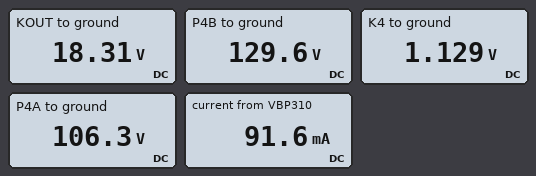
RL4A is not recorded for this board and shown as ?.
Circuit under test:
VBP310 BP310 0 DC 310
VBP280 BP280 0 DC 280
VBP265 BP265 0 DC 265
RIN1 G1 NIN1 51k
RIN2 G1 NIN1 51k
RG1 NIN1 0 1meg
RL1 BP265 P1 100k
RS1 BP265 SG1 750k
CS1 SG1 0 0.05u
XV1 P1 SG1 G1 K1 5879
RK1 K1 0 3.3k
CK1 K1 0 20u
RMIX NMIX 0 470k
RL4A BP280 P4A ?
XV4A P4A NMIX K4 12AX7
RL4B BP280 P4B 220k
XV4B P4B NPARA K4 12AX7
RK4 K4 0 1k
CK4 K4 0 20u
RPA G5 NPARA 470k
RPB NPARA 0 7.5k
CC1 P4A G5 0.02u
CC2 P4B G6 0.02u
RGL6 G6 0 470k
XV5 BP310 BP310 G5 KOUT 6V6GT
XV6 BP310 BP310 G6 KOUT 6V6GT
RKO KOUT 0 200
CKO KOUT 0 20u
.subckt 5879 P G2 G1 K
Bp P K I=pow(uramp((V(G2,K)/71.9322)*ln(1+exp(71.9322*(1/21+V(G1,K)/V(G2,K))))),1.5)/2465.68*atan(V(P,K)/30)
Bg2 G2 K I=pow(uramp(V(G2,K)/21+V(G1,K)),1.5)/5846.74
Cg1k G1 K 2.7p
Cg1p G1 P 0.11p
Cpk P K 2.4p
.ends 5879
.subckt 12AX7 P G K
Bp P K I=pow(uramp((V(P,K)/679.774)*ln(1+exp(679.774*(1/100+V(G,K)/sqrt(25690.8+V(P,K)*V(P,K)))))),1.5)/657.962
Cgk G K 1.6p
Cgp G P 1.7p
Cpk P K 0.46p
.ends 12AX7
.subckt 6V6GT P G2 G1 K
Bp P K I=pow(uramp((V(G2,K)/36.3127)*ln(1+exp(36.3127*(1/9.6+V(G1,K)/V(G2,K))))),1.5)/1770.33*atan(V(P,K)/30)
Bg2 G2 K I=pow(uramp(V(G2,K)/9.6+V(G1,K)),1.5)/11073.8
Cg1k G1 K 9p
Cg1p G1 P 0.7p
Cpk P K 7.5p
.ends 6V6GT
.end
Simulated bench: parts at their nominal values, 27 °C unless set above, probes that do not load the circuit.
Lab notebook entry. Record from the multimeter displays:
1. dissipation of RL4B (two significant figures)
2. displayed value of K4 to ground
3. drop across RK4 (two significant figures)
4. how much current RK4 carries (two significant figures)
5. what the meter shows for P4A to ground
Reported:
100 mW
1.129 V
1.1 V
1.1 mA
106.3 V
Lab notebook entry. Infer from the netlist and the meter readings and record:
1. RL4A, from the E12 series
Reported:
390 kΩ
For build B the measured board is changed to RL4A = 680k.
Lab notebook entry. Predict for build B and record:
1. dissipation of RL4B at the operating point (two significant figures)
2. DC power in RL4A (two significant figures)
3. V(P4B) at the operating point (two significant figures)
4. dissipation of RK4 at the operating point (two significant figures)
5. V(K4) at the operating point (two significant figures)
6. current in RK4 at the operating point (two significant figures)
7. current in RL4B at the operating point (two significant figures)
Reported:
110 mW
60 mW
120 V
1.0 mW
1.0 V
1.0 mA
720 µA
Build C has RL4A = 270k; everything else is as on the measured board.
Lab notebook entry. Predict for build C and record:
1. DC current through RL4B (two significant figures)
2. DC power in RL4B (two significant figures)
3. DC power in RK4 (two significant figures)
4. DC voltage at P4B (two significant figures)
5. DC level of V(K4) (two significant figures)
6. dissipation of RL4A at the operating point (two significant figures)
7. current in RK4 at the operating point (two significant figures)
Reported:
660 µA
95 mW
1.5 mW
140 V
1.2 V
86 mW
1.2 mA
